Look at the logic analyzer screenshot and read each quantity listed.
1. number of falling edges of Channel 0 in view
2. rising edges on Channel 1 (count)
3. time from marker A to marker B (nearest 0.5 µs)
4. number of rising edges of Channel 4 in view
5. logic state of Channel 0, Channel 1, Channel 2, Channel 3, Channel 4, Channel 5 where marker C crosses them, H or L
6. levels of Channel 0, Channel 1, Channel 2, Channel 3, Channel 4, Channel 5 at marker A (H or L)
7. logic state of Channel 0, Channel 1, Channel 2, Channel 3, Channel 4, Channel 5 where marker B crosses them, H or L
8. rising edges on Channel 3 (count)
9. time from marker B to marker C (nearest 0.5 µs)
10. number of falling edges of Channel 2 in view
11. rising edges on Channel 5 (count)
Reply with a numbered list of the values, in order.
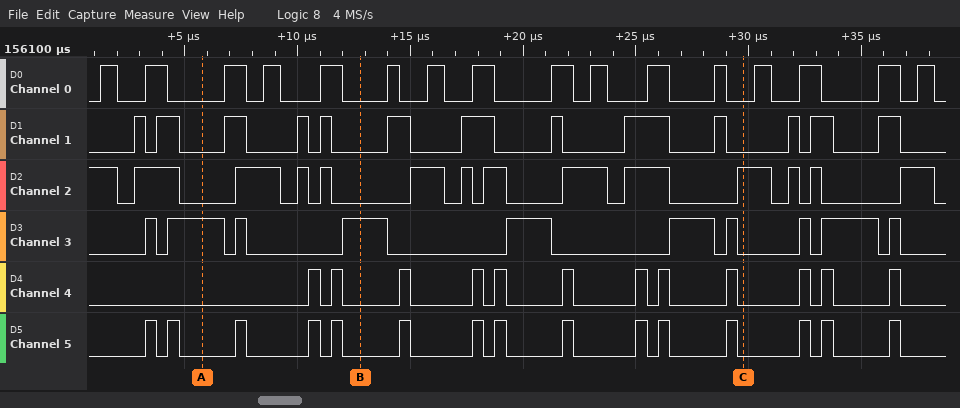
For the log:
1. 16
2. 13
3. 7 µs
4. 12
5. Channel 0=L, Channel 1=L, Channel 2=H, Channel 3=L, Channel 4=L, Channel 5=L
6. Channel 0=L, Channel 1=L, Channel 2=L, Channel 3=H, Channel 4=L, Channel 5=L
7. Channel 0=L, Channel 1=L, Channel 2=L, Channel 3=H, Channel 4=L, Channel 5=L
8. 10
9. 17 µs
10. 14
11. 15
